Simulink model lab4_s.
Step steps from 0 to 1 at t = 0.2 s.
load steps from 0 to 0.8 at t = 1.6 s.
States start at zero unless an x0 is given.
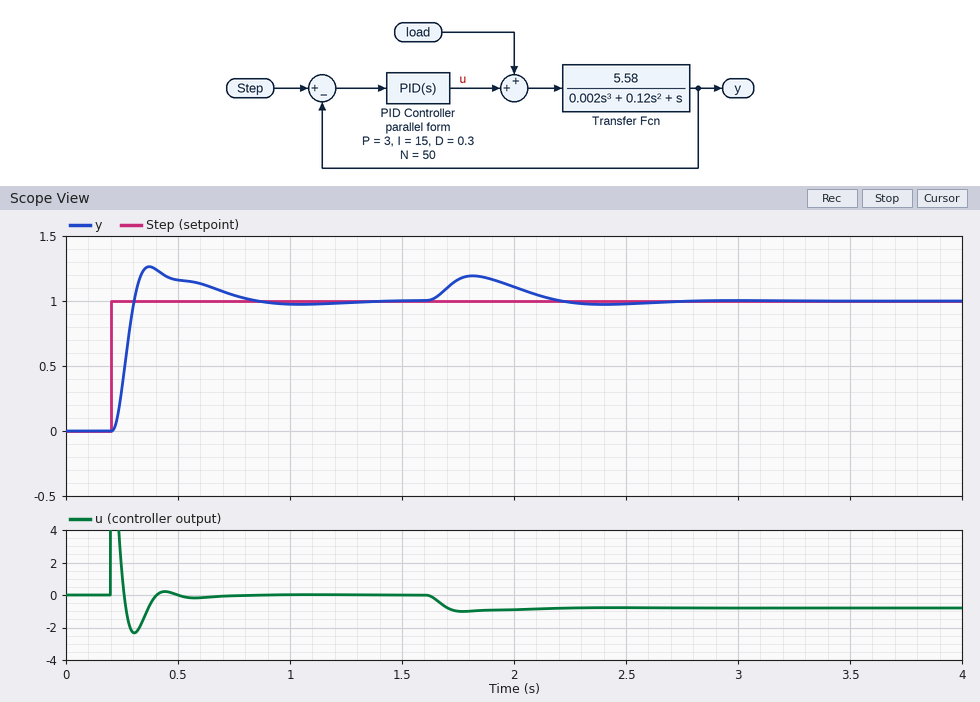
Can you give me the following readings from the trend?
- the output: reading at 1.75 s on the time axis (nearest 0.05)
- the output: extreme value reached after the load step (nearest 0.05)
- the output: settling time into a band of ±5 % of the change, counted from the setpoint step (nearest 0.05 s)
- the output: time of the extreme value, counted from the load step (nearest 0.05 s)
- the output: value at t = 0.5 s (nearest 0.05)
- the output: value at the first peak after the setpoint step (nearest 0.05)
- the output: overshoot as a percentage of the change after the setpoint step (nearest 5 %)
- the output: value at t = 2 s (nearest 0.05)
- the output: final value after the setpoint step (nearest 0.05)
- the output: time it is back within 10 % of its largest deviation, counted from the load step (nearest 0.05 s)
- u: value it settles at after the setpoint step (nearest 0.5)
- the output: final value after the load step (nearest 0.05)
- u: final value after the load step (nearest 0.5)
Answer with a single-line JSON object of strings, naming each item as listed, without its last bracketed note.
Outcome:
{"the output: reading at 1.75 s on the time axis": "1.15", "the output: extreme value reached after the load step": "1.20", "the output: settling time into a band of ±5 % of the change, counted from the setpoint step": "0.55 s", "the output: time of the extreme value, counted from the load step": "0.20 s", "the output: value at t = 0.5 s": "1.15", "the output: value at the first peak after the setpoint step": "1.25", "the output: overshoot as a percentage of the change after the setpoint step": "25 %", "the output: value at t = 2 s": "1.10", "the output: final value after the setpoint step": "1.00", "the output: time it is back within 10 % of its largest deviation, counted from the load step": "0.95 s", "u: value it settles at after the setpoint step": "0.0", "the output: final value after the load step": "1.00", "u: final value after the load step": "-1.0"}
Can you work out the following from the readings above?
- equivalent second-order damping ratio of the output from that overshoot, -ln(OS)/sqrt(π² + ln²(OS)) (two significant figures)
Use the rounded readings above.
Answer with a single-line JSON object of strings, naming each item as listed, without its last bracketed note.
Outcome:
{"equivalent second-order damping ratio of the output from that overshoot, -ln(OS)/sqrt(π² + ln²(OS))": "0.40"}
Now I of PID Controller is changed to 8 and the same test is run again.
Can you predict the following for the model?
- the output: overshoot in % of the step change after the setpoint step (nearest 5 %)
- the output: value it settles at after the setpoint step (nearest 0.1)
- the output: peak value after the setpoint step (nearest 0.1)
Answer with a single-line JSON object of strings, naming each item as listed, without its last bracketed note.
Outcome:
{"the output: overshoot in % of the step change after the setpoint step": "20 %", "the output: value it settles at after the setpoint step": "1.0", "the output: peak value after the setpoint step": "1.2"}
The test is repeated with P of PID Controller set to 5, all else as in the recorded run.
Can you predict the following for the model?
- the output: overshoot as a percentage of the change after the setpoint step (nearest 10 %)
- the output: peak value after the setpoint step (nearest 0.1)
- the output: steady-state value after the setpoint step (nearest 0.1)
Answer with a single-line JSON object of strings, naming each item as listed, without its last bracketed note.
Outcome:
{"the output: overshoot as a percentage of the change after the setpoint step": "40 %", "the output: peak value after the setpoint step": "1.4", "the output: steady-state value after the setpoint step": "1.0"}
